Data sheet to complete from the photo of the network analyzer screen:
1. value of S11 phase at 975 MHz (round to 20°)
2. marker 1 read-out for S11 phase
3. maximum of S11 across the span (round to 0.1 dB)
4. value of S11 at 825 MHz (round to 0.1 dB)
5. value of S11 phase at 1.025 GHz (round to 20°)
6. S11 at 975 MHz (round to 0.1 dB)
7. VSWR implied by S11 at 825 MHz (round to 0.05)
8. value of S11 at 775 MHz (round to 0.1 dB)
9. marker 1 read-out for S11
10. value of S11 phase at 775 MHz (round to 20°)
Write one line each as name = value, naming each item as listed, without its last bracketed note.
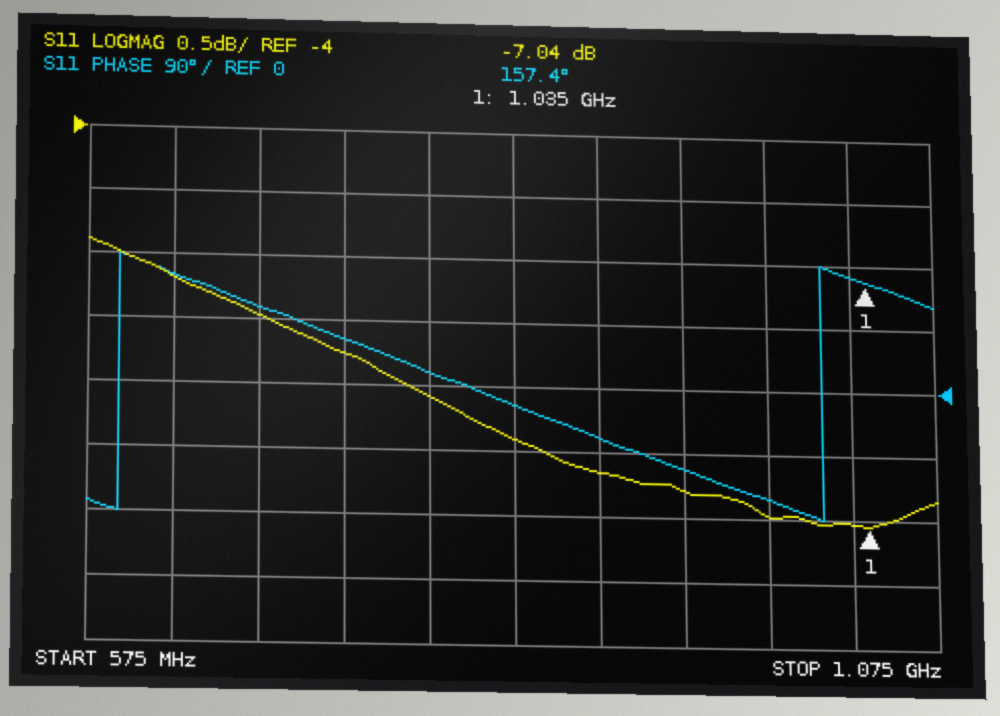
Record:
value of S11 phase at 975 MHz = -160°
marker 1 read-out for S11 phase = 157.4°
maximum of S11 across the span = -4.9 dB
value of S11 at 825 MHz = -6.4 dB
value of S11 phase at 1.025 GHz = 160°
S11 at 975 MHz = -7.0 dB
VSWR implied by S11 at 825 MHz = 2.85
value of S11 at 775 MHz = -6.1 dB
marker 1 read-out for S11 = -7.04 dB
value of S11 phase at 775 MHz = 20°
